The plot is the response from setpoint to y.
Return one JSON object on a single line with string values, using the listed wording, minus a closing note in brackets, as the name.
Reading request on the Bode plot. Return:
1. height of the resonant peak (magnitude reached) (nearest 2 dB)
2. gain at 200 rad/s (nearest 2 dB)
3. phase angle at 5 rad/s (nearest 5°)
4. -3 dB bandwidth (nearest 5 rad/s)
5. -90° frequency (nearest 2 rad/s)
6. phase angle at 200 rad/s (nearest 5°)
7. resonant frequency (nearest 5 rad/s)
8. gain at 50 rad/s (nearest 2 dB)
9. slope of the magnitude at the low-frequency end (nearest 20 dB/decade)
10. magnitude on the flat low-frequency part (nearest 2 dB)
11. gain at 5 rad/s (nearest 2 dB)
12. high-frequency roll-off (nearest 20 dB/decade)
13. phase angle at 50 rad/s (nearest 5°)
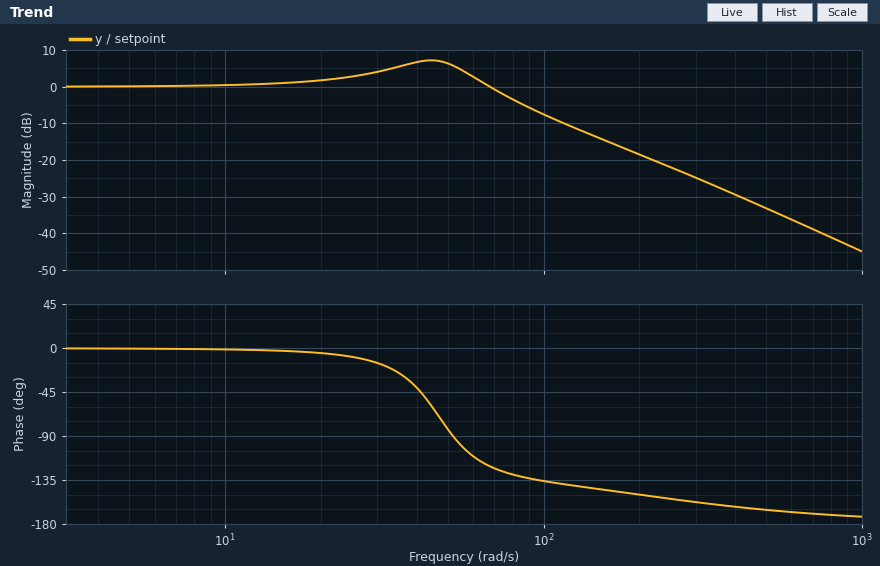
{"height of the resonant peak (magnitude reached)": "8 dB", "gain at 200 rad/s": "-18 dB", "phase angle at 5 rad/s": "0°", "-3 dB bandwidth": "80 rad/s", "-90° frequency": "52 rad/s", "phase angle at 200 rad/s": "-150°", "resonant frequency": "45 rad/s", "gain at 50 rad/s": "6 dB", "slope of the magnitude at the low-frequency end": "0 dB/decade", "magnitude on the flat low-frequency part": "0 dB", "gain at 5 rad/s": "0 dB", "high-frequency roll-off": "-40 dB/decade", "phase angle at 50 rad/s": "-85°"}
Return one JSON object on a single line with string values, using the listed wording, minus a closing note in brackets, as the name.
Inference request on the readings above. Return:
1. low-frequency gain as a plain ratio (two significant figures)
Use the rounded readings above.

{"low-frequency gain as a plain ratio": "1.0"}
